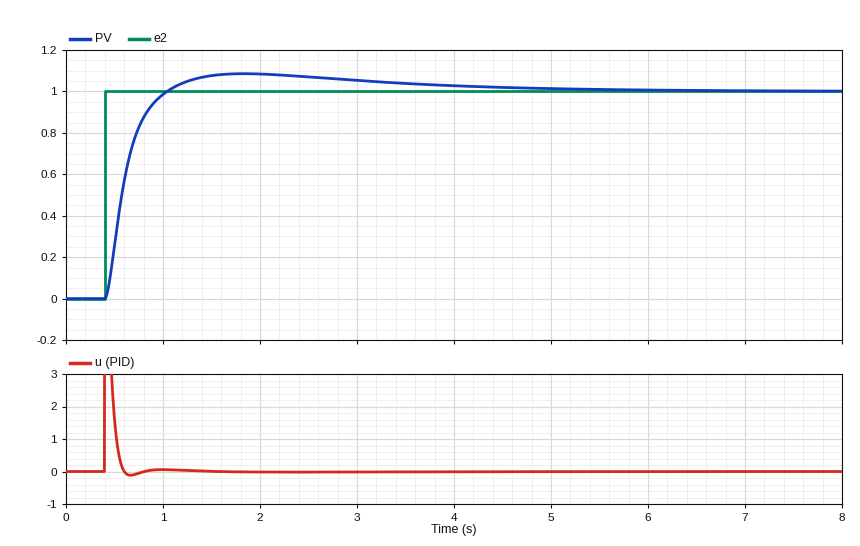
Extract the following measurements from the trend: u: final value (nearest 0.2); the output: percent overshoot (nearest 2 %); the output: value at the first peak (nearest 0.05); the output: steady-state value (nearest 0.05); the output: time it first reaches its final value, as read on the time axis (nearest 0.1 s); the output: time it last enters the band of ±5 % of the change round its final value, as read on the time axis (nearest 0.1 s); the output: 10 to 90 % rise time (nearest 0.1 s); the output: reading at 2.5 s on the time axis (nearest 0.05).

0.0
8 %
1.10
1.00
1.0 s
3.1 s
0.4 s
1.05
